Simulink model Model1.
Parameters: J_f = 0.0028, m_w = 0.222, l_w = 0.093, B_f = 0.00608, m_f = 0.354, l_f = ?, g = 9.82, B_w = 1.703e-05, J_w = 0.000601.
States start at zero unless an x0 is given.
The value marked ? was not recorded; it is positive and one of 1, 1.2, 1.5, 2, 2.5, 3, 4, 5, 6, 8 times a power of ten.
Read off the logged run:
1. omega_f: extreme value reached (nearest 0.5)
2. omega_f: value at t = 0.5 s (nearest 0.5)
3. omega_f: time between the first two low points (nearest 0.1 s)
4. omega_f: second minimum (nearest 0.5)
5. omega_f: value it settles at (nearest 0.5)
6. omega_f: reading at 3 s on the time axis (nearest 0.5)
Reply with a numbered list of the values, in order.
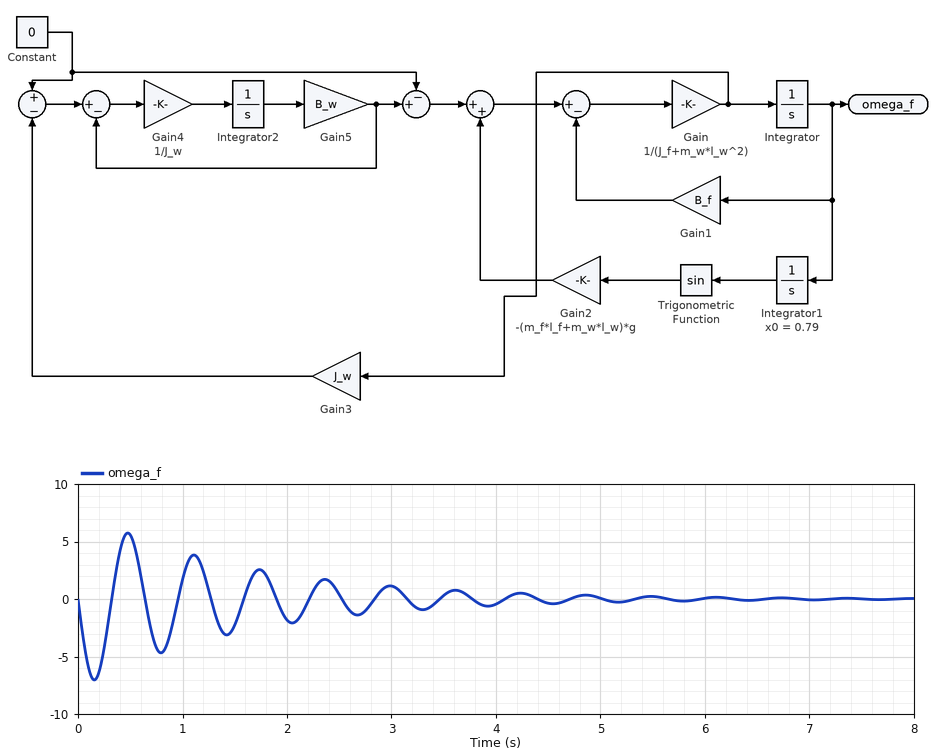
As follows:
1. -7.0
2. 5.5
3. 0.6 s
4. -4.5
5. 0.0
6. 1.0
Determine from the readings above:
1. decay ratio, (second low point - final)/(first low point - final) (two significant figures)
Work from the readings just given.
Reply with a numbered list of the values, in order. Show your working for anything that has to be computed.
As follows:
1. (-4.5 - 0) / (-7 - 0) = 0.64
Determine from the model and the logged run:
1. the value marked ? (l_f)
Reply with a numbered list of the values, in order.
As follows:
1. 0.08
